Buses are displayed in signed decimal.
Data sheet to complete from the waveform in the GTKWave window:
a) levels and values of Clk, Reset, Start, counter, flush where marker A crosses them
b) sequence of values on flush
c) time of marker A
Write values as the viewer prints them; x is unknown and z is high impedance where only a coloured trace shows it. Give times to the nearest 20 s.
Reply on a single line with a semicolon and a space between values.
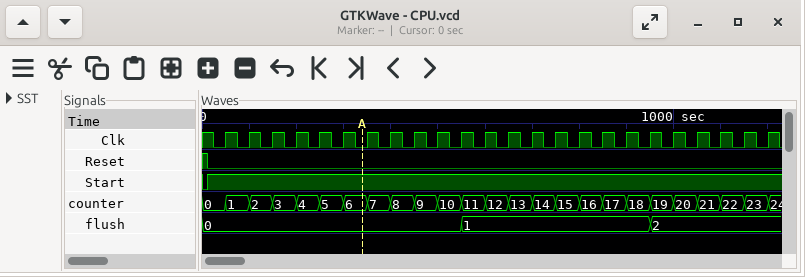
Clk=0, Reset=0, Start=1, counter=6, flush=0; 0, 1, 2; 340 s
